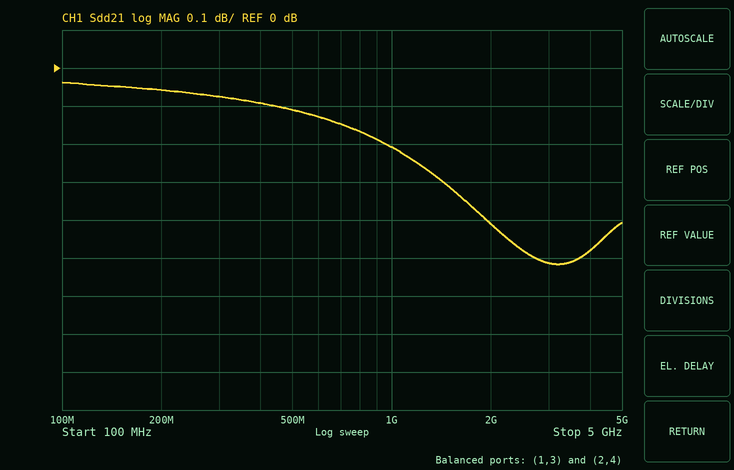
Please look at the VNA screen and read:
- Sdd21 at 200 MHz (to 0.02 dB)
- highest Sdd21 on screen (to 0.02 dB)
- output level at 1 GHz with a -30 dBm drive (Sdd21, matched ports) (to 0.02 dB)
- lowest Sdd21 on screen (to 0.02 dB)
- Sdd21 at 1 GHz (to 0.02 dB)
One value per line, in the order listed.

-0.06 dB
-0.04 dB
-30.20 dBm
-0.52 dB
-0.20 dB
